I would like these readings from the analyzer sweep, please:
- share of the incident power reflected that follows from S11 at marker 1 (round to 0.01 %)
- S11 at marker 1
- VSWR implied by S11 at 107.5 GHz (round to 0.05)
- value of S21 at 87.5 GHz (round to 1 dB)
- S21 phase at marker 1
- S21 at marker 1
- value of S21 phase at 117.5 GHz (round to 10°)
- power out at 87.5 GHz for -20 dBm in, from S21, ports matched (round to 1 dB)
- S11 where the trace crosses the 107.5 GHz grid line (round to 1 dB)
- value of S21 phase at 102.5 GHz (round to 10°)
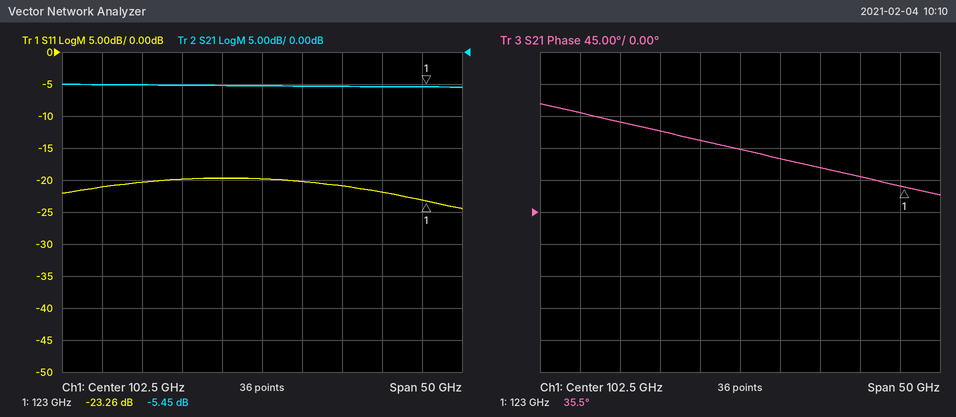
0.47 %
-23.26 dB
1.20
-5 dB
35.5°
-5.45 dB
50°
-25 dBm
-20 dB
90°
